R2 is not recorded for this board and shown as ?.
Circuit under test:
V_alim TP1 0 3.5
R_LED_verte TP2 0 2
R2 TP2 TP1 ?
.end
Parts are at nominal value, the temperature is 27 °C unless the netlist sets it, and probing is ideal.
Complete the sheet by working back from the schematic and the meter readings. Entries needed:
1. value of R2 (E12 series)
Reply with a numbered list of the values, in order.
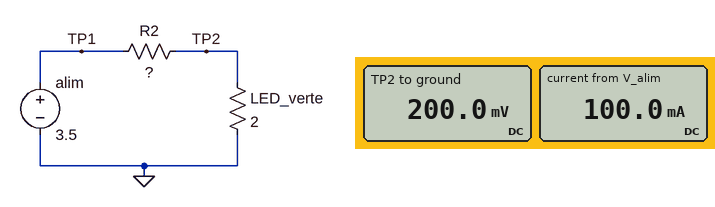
1. 33 Ω
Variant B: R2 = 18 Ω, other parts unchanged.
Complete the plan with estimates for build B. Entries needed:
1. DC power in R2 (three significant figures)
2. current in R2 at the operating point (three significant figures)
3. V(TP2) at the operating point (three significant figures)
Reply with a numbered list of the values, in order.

1. 551 mW
2. 175 mA
3. 350 mV
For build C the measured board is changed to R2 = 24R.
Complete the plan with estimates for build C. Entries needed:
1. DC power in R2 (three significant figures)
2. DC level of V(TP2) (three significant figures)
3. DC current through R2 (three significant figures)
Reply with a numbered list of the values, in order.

1. 435 mW
2. 269 mV
3. 135 mA
